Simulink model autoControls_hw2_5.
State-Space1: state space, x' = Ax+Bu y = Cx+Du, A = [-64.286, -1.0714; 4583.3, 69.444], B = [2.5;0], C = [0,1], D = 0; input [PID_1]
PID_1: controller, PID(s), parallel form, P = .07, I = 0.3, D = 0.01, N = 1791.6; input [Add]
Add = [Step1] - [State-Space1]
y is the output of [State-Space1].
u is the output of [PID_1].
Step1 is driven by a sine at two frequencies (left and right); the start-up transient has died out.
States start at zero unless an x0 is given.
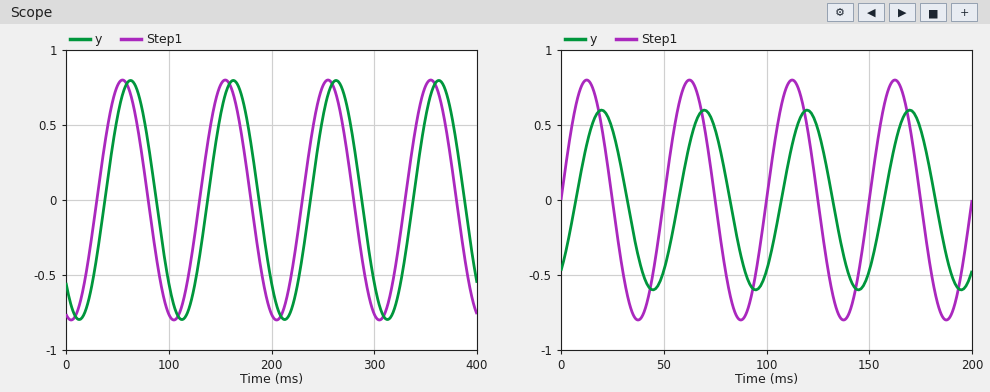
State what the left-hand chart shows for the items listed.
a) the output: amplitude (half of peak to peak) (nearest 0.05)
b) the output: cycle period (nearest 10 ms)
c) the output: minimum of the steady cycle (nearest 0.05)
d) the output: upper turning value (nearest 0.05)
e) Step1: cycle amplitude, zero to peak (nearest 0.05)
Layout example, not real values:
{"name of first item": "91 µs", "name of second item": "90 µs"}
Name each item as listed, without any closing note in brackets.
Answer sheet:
{"the output: amplitude (half of peak to peak)": "0.80", "the output: cycle period": "100 ms", "the output: minimum of the steady cycle": "-0.80", "the output: upper turning value": "0.80", "Step1: cycle amplitude, zero to peak": "0.80"}
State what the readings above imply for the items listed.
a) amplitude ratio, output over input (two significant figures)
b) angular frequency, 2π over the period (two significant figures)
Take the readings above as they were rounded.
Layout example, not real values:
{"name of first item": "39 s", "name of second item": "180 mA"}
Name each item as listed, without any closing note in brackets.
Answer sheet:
{"amplitude ratio, output over input": "1.0", "angular frequency, 2π over the period": "0.063 rad/ms"}
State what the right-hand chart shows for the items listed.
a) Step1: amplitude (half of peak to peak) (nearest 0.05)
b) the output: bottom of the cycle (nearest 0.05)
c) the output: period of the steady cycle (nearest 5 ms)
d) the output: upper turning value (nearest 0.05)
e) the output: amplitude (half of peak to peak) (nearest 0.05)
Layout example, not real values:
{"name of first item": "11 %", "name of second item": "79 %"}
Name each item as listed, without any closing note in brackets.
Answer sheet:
{"Step1: amplitude (half of peak to peak)": "0.80", "the output: bottom of the cycle": "-0.60", "the output: period of the steady cycle": "50 ms", "the output: upper turning value": "0.60", "the output: amplitude (half of peak to peak)": "0.60"}
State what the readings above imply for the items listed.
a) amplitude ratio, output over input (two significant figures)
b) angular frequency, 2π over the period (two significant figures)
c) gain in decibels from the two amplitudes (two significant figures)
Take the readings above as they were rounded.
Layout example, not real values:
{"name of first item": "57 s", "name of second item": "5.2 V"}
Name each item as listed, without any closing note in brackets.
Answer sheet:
{"amplitude ratio, output over input": "0.75", "angular frequency, 2π over the period": "0.13 rad/ms", "gain in decibels from the two amplitudes": "-2.5 dB"}
